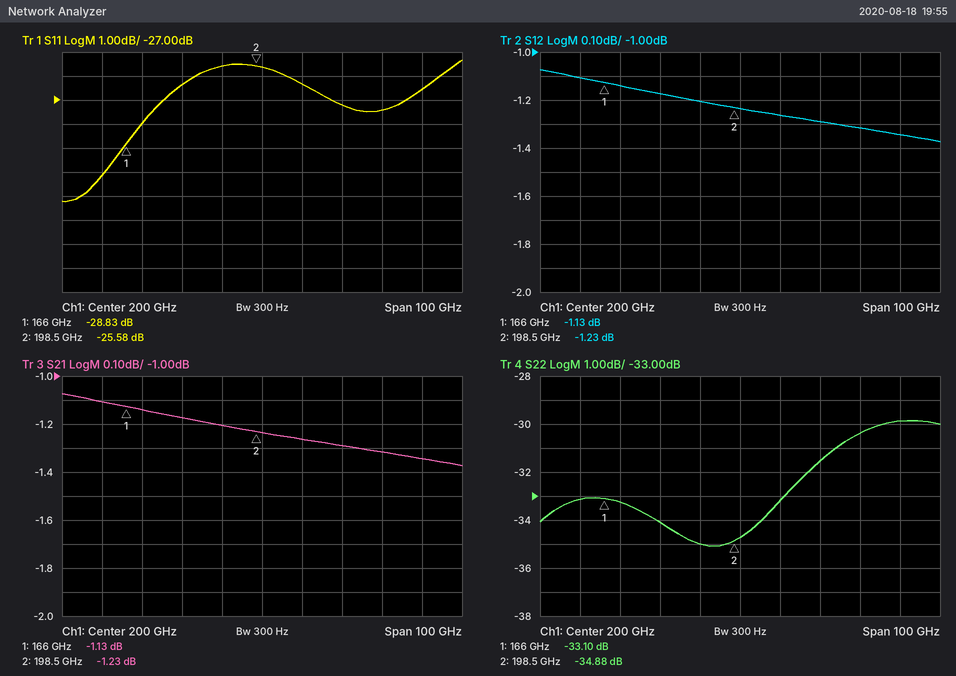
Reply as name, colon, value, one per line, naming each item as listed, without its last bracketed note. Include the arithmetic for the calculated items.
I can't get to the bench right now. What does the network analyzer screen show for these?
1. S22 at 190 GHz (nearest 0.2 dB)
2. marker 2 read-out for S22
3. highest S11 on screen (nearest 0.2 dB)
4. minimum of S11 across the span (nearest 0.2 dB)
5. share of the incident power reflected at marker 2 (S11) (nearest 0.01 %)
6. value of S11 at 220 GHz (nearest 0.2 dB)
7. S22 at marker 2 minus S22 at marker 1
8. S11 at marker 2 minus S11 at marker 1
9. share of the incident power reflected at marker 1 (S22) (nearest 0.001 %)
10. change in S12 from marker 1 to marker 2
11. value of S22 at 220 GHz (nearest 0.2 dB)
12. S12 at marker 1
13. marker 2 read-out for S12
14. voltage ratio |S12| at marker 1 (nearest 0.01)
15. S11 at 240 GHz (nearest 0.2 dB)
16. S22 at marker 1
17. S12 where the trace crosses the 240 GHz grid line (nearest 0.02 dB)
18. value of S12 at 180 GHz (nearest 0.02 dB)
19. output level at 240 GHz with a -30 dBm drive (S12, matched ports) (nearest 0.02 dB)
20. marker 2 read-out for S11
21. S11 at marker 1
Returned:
S22 at 190 GHz: -35.0 dB
marker 2 read-out for S22: -34.88 dB
highest S11 on screen: -25.4 dB
minimum of S11 across the span: -31.2 dB
share of the incident power reflected at marker 2 (S11): 10^(-25.58/10) ≈ 0.28 %
value of S11 at 220 GHz: -27.2 dB
S22 at marker 2 minus S22 at marker 1: -34.88 − (-33.1) = -1.78 dB
S11 at marker 2 minus S11 at marker 1: -25.58 − (-28.83) = 3.25 dB
share of the incident power reflected at marker 1 (S22): 10^(-33.1/10) ≈ 0.049 %
change in S12 from marker 1 to marker 2: -1.23 − (-1.13) = -0.10 dB
value of S22 at 220 GHz: -31.6 dB
S12 at marker 1: -1.13 dB
marker 2 read-out for S12: -1.23 dB
voltage ratio |S12| at marker 1: 10^(-1.13/20) ≈ 0.88
S11 at 240 GHz: -26.6 dB
S22 at marker 1: -33.10 dB
S12 where the trace crosses the 240 GHz grid line: -1.34 dB
value of S12 at 180 GHz: -1.18 dB
output level at 240 GHz with a -30 dBm drive (S12, matched ports): -30 dBm + (-1.34 dB) = -31.34 dBm
marker 2 read-out for S11: -25.58 dB
S11 at marker 1: -28.83 dB
